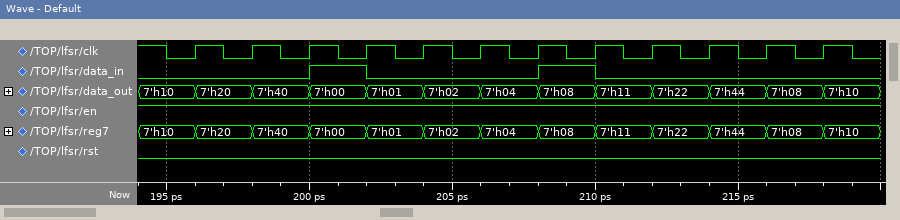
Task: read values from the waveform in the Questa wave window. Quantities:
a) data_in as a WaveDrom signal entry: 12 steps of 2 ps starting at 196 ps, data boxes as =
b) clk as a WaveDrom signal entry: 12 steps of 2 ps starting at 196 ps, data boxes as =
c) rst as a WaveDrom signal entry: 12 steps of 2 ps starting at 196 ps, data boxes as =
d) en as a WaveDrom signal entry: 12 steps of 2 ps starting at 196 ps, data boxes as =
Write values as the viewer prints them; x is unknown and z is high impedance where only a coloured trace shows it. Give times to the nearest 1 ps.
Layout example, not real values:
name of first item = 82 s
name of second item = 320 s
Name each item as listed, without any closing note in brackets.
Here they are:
data_in as a WaveDrom signal entry: 12 steps of 2 ps starting at 196 ps, data boxes as = = {name: 'data_in', wave: '0.10..10....'}
clk as a WaveDrom signal entry: 12 steps of 2 ps starting at 196 ps, data boxes as = = {name: 'clk', wave: 'p...........'}
rst as a WaveDrom signal entry: 12 steps of 2 ps starting at 196 ps, data boxes as = = {name: 'rst', wave: '0...........'}
en as a WaveDrom signal entry: 12 steps of 2 ps starting at 196 ps, data boxes as = = {name: 'en', wave: '1...........'}
